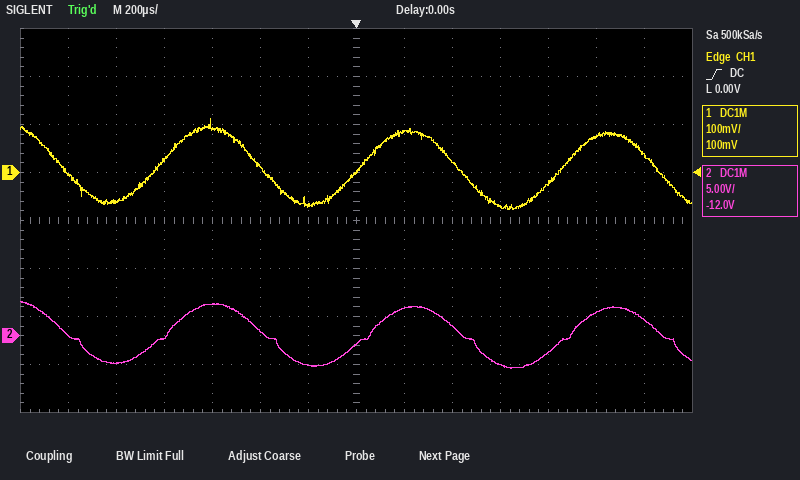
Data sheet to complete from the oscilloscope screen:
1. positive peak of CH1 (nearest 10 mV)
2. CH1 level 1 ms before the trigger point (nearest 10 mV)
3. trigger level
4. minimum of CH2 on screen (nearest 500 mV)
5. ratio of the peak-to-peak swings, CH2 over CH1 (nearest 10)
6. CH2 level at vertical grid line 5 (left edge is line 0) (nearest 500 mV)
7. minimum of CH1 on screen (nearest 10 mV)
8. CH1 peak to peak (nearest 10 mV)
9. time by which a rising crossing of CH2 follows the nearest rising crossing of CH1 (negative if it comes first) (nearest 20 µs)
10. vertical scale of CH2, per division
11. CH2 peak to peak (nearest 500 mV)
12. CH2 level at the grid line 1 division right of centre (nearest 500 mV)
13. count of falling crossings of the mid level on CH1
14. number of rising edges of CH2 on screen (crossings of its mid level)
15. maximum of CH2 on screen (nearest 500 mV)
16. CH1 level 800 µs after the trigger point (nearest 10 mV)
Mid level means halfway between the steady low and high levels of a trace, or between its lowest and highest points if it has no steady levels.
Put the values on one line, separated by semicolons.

110 mV; -60 mV; 0.00 V; -3.5 V; 40; 500 mV; -80 mV; 190 mV; +20 µs; 5 V; 7.0 V; 3.0 V; 4; 3; 3.5 V; -20 mV
